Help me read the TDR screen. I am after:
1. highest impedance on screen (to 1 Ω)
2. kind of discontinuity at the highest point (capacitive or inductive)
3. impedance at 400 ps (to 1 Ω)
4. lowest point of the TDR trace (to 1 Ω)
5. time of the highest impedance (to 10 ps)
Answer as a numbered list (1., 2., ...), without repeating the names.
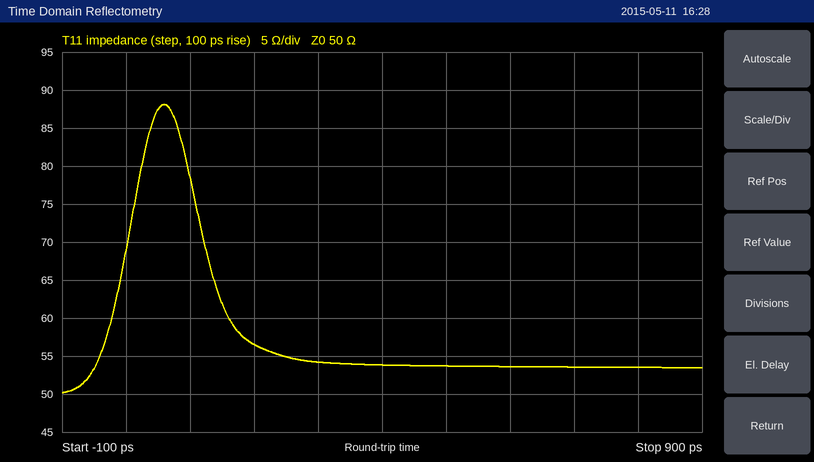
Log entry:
1. 88 Ω
2. inductive
3. 54 Ω
4. 50 Ω
5. 60 ps
